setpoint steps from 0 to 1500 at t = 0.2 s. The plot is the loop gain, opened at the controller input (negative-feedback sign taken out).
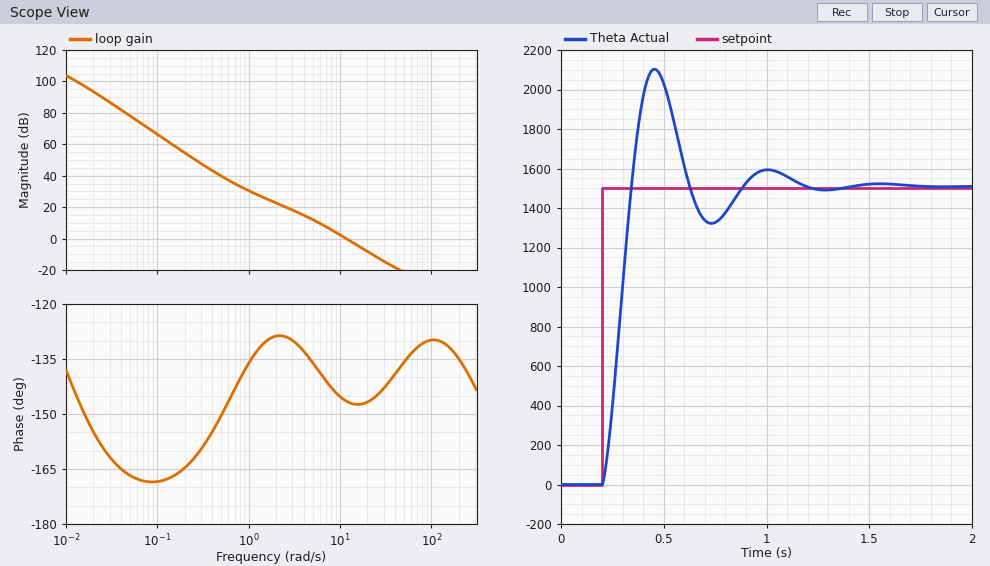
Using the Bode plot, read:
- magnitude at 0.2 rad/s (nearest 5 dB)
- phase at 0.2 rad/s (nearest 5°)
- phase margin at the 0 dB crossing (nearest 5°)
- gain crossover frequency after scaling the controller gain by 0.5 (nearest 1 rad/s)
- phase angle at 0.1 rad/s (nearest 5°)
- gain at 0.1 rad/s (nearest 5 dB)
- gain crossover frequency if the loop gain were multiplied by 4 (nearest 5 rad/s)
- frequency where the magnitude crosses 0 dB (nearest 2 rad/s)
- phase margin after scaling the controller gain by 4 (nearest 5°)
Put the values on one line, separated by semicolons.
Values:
55 dB; -165°; 35°; 8 rad/s; -170°; 65 dB; 25 rad/s; 12 rad/s; 35°
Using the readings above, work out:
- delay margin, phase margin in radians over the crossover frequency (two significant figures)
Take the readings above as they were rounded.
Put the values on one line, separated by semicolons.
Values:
0.051 s
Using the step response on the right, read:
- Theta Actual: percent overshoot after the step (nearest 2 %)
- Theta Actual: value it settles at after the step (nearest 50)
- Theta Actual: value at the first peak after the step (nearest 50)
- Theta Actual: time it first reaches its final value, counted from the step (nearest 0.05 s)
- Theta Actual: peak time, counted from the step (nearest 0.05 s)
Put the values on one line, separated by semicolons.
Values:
40 %; 1500; 2100; 0.15 s; 0.25 s
